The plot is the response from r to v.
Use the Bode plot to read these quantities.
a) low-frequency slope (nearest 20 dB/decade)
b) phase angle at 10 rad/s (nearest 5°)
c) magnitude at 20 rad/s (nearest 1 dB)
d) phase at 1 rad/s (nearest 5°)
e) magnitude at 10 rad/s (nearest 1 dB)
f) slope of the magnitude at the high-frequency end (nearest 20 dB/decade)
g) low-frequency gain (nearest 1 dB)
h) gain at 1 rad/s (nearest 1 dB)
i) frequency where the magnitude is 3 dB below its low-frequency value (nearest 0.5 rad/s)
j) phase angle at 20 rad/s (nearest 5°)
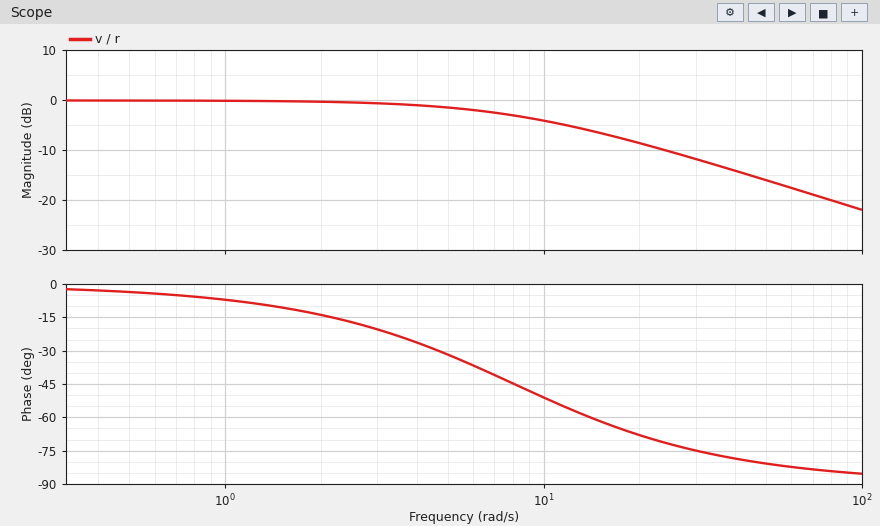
0 dB/decade
-50°
-9 dB
-5°
-4 dB
-20 dB/decade
0 dB
0 dB
8.0 rad/s
-70°
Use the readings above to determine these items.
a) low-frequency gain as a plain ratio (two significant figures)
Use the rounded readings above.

1.0
